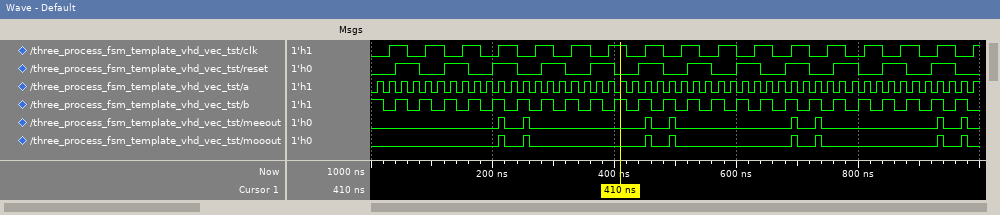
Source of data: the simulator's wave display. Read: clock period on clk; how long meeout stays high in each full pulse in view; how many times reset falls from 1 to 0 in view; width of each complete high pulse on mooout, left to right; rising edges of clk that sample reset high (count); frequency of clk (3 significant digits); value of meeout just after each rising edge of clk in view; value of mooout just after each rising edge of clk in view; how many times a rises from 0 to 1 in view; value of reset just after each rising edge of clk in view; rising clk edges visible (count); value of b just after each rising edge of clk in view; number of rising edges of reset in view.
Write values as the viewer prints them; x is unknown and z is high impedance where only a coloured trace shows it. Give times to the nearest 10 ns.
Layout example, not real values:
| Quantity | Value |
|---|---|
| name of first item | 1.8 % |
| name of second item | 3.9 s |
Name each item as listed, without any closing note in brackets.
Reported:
| Quantity | Value |
|---|---|
| clock period on clk | 60 ns |
| how long meeout stays high in each full pulse in view | 10 ns, 10 ns, 10 ns, 10 ns, 10 ns, 10 ns, 10 ns, 10 ns |
| how many times reset falls from 1 to 0 in view | 12 |
| width of each complete high pulse on mooout, left to right | 10 ns, 10 ns, 10 ns, 10 ns, 10 ns, 10 ns, 10 ns, 10 ns |
| rising edges of clk that sample reset high | 8 |
| frequency of clk | 16.7 MHz |
| value of meeout just after each rising edge of clk in view | 0 0 0 1 0 0 0 1 0 0 0 1 0 0 0 1 0 |
| value of mooout just after each rising edge of clk in view | 0 0 0 1 0 0 0 1 0 0 0 1 0 0 0 1 0 |
| how many times a rises from 0 to 1 in view | 50 |
| value of reset just after each rising edge of clk in view | 0 0 1 1 0 0 1 1 0 0 1 1 0 0 1 1 0 |
| rising clk edges visible | 17 |
| value of b just after each rising edge of clk in view | 0 1 0 1 0 1 0 1 0 1 0 1 0 1 0 1 0 |
| number of rising edges of reset in view | 12 |
